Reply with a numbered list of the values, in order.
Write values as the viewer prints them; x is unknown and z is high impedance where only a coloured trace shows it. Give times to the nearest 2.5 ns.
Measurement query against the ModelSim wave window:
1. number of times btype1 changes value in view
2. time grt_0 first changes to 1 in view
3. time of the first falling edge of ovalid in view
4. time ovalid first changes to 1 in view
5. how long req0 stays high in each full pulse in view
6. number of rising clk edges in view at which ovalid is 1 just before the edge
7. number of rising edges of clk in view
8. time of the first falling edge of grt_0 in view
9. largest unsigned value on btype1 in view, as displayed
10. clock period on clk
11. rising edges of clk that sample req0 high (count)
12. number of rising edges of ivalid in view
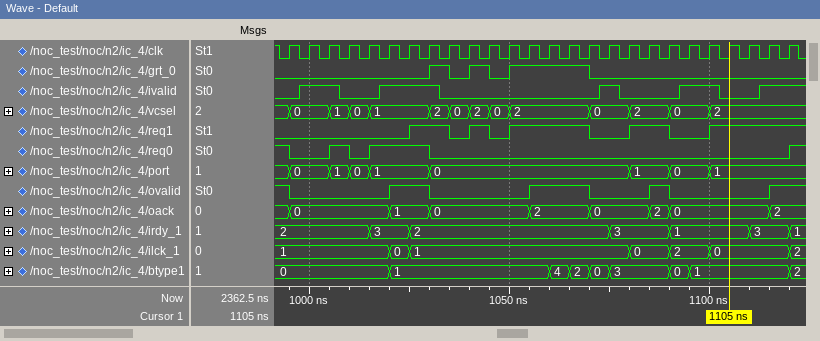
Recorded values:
1. 8
2. 1030 ns
3. 995 ns
4. 1020 ns
5. 5 ns, 15 ns
6. 8
7. 26
8. 1035 ns
9. 4
10. 5 ns
11. 5
12. 5
